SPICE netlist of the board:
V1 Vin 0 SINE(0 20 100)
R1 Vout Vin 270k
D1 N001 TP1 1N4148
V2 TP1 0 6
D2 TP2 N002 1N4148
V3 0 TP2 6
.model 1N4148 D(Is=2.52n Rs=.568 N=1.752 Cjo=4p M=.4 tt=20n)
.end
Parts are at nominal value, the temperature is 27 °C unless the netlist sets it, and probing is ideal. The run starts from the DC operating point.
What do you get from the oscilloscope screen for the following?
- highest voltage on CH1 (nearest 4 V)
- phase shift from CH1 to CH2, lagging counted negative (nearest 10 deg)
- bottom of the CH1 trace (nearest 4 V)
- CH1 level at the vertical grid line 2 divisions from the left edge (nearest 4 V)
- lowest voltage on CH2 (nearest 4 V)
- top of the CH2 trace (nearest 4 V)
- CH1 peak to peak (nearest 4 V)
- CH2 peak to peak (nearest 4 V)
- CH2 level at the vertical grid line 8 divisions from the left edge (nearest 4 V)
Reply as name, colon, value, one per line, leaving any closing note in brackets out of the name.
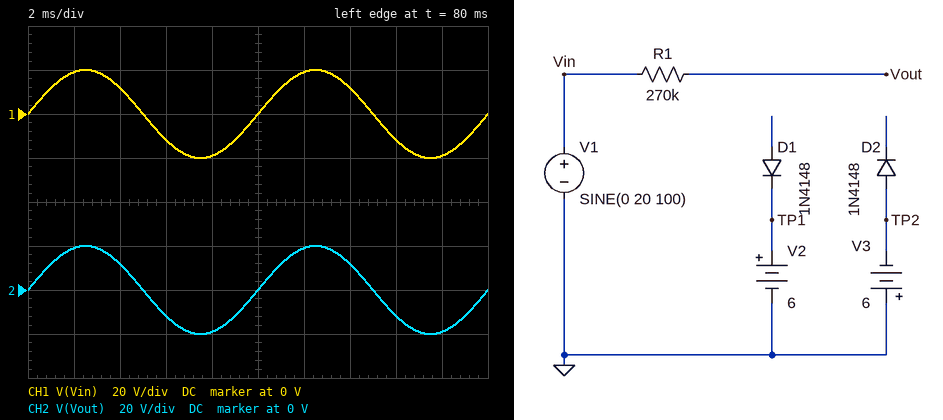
highest voltage on CH1: 20 V
phase shift from CH1 to CH2, lagging counted negative: 0 deg
bottom of the CH1 trace: -20 V
CH1 level at the vertical grid line 2 divisions from the left edge: 12 V
lowest voltage on CH2: -20 V
top of the CH2 trace: 20 V
CH1 peak to peak: 40 V
CH2 peak to peak: 40 V
CH2 level at the vertical grid line 8 divisions from the left edge: -12 V
